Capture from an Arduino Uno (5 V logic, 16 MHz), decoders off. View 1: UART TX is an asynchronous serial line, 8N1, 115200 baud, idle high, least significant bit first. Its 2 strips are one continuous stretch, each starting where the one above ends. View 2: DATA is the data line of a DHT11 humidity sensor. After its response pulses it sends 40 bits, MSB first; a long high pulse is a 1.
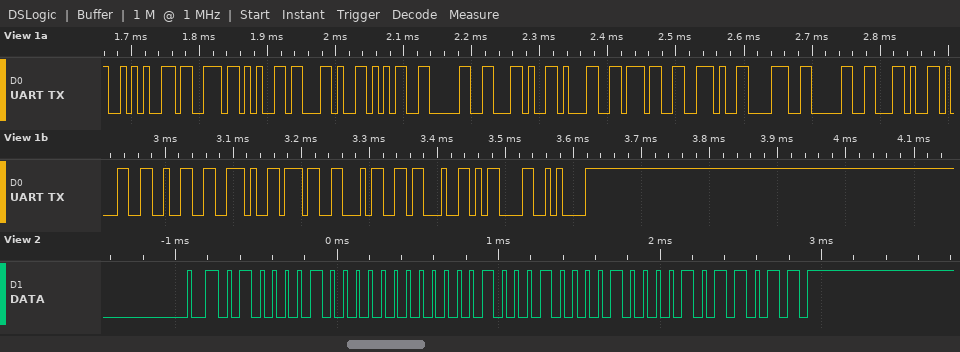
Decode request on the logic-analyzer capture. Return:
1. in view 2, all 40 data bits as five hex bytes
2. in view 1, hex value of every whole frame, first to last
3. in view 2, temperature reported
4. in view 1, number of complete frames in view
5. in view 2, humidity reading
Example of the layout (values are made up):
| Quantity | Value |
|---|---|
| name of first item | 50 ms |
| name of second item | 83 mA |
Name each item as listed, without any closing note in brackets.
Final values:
| Quantity | Value |
|---|---|
| in view 2, all 40 data bits as five hex bytes | 42 00 11 08 5B |
| in view 1, hex value of every whole frame, first to last | 2A 73 65 2C 35 30 2C 31 37 2E 38 30 2C 31 32 2E 37 34 23 0D 0A |
| in view 2, temperature reported | 17.8 °C |
| in view 1, number of complete frames in view | 21 |
| in view 2, humidity reading | 66 % |
